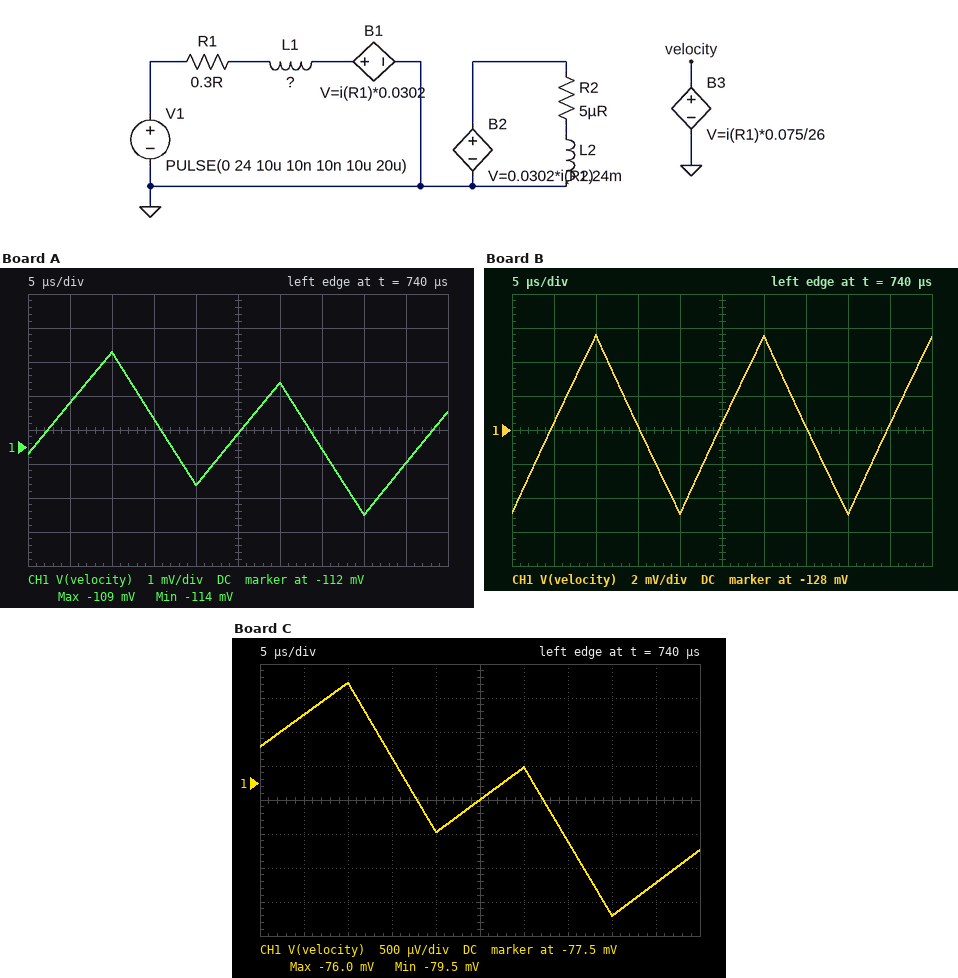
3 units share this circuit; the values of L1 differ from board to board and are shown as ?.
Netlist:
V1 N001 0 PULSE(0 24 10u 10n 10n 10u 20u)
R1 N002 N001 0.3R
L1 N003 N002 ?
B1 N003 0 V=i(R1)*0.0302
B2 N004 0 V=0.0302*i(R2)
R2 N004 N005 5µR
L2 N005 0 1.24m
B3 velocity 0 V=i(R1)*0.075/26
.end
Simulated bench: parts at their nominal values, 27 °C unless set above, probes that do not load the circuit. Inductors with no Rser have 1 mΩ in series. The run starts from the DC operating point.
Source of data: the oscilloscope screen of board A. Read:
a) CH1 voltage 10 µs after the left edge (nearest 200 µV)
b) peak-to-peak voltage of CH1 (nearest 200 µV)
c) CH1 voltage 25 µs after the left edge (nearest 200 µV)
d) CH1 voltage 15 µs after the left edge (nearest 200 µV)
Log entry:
-109.2 mV
4.8 mV
-111.6 mV
-111.2 mV
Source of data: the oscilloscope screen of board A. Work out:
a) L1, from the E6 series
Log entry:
100 µH
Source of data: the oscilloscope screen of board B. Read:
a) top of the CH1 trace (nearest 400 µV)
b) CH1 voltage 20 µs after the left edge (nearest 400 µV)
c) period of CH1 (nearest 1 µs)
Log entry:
-122.4 mV
-132.8 mV
20 µs
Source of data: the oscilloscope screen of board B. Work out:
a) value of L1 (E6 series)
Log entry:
33 µH
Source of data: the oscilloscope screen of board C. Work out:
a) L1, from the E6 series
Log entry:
220 µH
